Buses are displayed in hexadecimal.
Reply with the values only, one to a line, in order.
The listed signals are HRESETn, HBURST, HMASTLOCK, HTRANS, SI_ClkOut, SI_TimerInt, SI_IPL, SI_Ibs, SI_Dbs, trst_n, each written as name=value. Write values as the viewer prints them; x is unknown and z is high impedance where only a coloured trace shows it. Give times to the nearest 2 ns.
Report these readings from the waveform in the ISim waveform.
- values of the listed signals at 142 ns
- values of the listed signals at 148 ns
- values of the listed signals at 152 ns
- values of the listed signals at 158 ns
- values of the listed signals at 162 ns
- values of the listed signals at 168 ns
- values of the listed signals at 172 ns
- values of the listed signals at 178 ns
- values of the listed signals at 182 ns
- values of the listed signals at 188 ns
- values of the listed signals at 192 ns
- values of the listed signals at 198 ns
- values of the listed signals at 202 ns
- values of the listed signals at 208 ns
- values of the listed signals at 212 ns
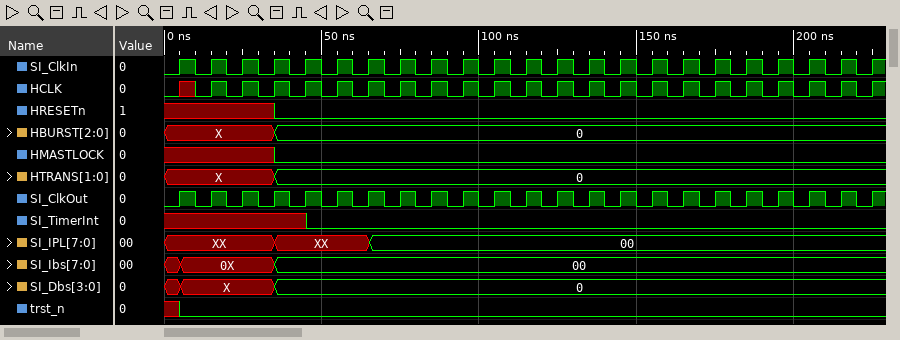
HRESETn=0, HBURST=0, HMASTLOCK=0, HTRANS=0, SI_ClkOut=0, SI_TimerInt=0, SI_IPL=00, SI_Ibs=00, SI_Dbs=0, trst_n=0
HRESETn=0, HBURST=0, HMASTLOCK=0, HTRANS=0, SI_ClkOut=1, SI_TimerInt=0, SI_IPL=00, SI_Ibs=00, SI_Dbs=0, trst_n=0
HRESETn=0, HBURST=0, HMASTLOCK=0, HTRANS=0, SI_ClkOut=0, SI_TimerInt=0, SI_IPL=00, SI_Ibs=00, SI_Dbs=0, trst_n=0
HRESETn=0, HBURST=0, HMASTLOCK=0, HTRANS=0, SI_ClkOut=1, SI_TimerInt=0, SI_IPL=00, SI_Ibs=00, SI_Dbs=0, trst_n=0
HRESETn=0, HBURST=0, HMASTLOCK=0, HTRANS=0, SI_ClkOut=0, SI_TimerInt=0, SI_IPL=00, SI_Ibs=00, SI_Dbs=0, trst_n=0
HRESETn=0, HBURST=0, HMASTLOCK=0, HTRANS=0, SI_ClkOut=1, SI_TimerInt=0, SI_IPL=00, SI_Ibs=00, SI_Dbs=0, trst_n=0
HRESETn=0, HBURST=0, HMASTLOCK=0, HTRANS=0, SI_ClkOut=0, SI_TimerInt=0, SI_IPL=00, SI_Ibs=00, SI_Dbs=0, trst_n=0
HRESETn=0, HBURST=0, HMASTLOCK=0, HTRANS=0, SI_ClkOut=1, SI_TimerInt=0, SI_IPL=00, SI_Ibs=00, SI_Dbs=0, trst_n=0
HRESETn=0, HBURST=0, HMASTLOCK=0, HTRANS=0, SI_ClkOut=0, SI_TimerInt=0, SI_IPL=00, SI_Ibs=00, SI_Dbs=0, trst_n=0
HRESETn=0, HBURST=0, HMASTLOCK=0, HTRANS=0, SI_ClkOut=1, SI_TimerInt=0, SI_IPL=00, SI_Ibs=00, SI_Dbs=0, trst_n=0
HRESETn=0, HBURST=0, HMASTLOCK=0, HTRANS=0, SI_ClkOut=0, SI_TimerInt=0, SI_IPL=00, SI_Ibs=00, SI_Dbs=0, trst_n=0
HRESETn=0, HBURST=0, HMASTLOCK=0, HTRANS=0, SI_ClkOut=1, SI_TimerInt=0, SI_IPL=00, SI_Ibs=00, SI_Dbs=0, trst_n=0
HRESETn=0, HBURST=0, HMASTLOCK=0, HTRANS=0, SI_ClkOut=0, SI_TimerInt=0, SI_IPL=00, SI_Ibs=00, SI_Dbs=0, trst_n=0
HRESETn=0, HBURST=0, HMASTLOCK=0, HTRANS=0, SI_ClkOut=1, SI_TimerInt=0, SI_IPL=00, SI_Ibs=00, SI_Dbs=0, trst_n=0
HRESETn=0, HBURST=0, HMASTLOCK=0, HTRANS=0, SI_ClkOut=0, SI_TimerInt=0, SI_IPL=00, SI_Ibs=00, SI_Dbs=0, trst_n=0
